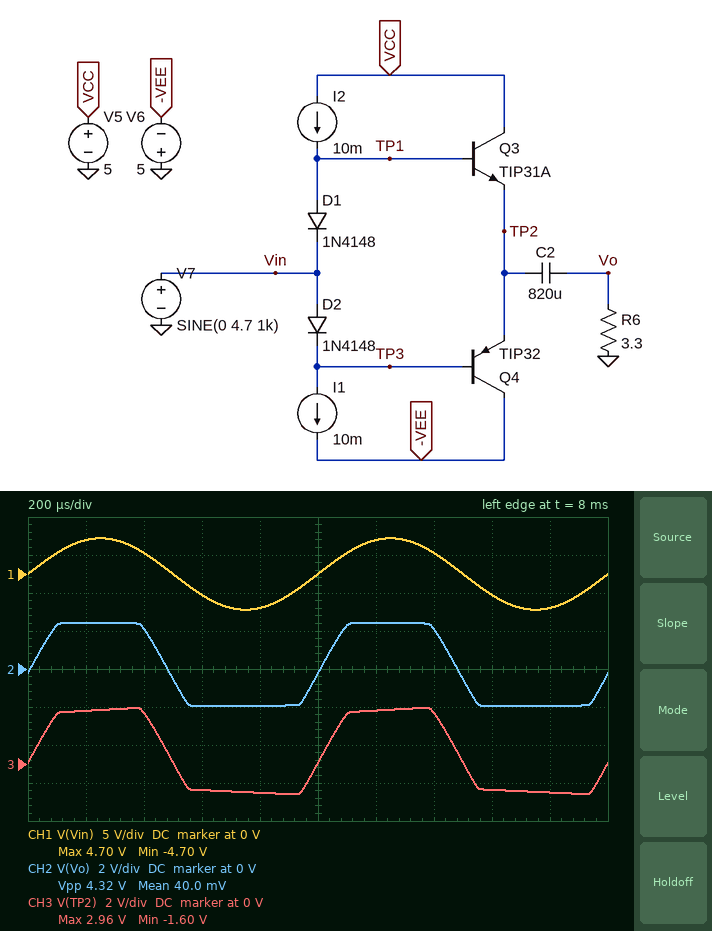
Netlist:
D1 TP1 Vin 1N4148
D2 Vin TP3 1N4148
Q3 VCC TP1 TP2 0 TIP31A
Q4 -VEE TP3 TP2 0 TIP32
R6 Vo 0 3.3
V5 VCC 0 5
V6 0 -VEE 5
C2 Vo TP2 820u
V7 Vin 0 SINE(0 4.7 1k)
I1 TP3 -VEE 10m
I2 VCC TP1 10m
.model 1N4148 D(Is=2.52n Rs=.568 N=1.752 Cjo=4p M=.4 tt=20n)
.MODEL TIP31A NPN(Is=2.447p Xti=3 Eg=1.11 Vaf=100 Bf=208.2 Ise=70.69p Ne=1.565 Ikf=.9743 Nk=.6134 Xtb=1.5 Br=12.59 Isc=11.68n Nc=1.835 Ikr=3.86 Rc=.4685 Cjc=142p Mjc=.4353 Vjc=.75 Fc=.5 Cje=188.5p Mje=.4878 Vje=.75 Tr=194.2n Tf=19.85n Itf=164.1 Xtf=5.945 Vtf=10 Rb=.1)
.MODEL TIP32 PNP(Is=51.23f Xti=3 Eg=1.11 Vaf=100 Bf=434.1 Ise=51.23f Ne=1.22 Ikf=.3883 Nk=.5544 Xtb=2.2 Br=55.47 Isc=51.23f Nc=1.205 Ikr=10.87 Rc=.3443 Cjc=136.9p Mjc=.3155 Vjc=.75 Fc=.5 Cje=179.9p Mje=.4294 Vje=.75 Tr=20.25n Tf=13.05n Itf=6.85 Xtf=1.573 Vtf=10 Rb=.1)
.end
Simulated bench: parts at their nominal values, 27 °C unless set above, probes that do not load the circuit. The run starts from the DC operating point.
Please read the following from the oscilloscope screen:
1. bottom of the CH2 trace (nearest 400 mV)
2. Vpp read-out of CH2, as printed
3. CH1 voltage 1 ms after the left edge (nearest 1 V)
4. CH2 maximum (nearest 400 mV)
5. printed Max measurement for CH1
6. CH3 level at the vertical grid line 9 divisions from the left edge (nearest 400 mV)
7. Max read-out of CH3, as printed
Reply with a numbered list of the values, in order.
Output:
1. -2.0 V
2. 4.32 V
3. 0 V
4. 2.4 V
5. 4.70 V
6. -1.6 V
7. 2.96 V
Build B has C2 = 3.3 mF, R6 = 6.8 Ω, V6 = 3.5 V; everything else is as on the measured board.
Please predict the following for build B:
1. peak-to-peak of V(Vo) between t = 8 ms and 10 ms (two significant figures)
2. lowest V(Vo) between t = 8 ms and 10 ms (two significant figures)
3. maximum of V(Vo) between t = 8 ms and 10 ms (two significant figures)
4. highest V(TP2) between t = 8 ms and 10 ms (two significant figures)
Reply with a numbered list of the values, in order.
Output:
1. 7.8 V
2. -3.4 V
3. 4.4 V
4. 4.5 V
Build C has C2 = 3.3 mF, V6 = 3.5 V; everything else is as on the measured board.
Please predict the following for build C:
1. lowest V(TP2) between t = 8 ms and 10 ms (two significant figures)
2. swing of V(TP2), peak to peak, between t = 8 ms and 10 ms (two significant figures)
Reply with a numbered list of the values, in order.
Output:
1. -1.7 V
2. 4.4 V
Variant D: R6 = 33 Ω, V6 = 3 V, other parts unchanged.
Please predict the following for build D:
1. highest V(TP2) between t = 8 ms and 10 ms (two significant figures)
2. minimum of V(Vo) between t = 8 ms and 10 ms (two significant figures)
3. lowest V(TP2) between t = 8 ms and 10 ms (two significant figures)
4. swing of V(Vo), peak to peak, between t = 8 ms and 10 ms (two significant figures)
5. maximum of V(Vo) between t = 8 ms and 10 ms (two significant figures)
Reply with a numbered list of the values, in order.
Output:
1. 4.7 V
2. -3.1 V
3. -3.0 V
4. 7.7 V
5. 4.6 V
